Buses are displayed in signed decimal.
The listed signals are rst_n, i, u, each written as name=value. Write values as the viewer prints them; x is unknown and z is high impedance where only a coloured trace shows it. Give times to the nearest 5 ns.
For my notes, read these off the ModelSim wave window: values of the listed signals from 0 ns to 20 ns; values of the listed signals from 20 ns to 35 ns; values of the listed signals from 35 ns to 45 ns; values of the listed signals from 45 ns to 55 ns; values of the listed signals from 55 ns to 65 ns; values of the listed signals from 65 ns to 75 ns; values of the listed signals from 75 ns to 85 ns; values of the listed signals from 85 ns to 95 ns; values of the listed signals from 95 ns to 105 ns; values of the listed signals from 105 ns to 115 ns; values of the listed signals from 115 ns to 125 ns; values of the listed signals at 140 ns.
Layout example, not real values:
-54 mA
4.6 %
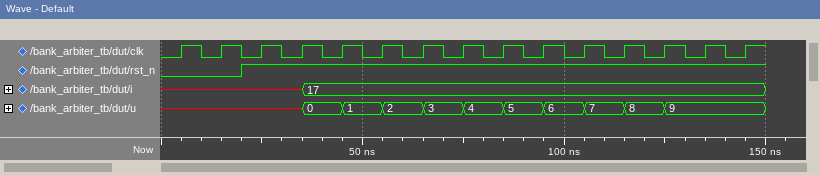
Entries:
rst_n=0, i=x, u=x
rst_n=1, i=x, u=x
rst_n=1, i=17, u=0
rst_n=1, i=17, u=1
rst_n=1, i=17, u=2
rst_n=1, i=17, u=3
rst_n=1, i=17, u=4
rst_n=1, i=17, u=5
rst_n=1, i=17, u=6
rst_n=1, i=17, u=7
rst_n=1, i=17, u=8
rst_n=1, i=17, u=9
